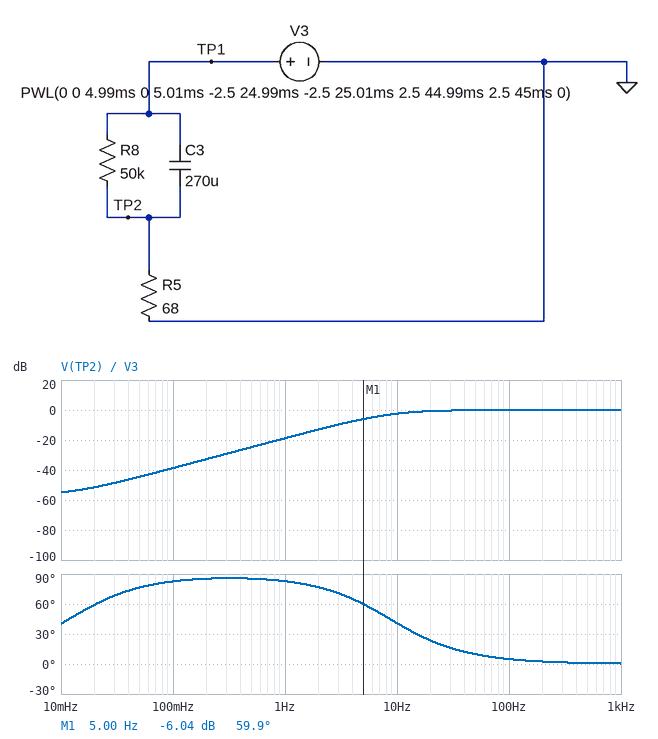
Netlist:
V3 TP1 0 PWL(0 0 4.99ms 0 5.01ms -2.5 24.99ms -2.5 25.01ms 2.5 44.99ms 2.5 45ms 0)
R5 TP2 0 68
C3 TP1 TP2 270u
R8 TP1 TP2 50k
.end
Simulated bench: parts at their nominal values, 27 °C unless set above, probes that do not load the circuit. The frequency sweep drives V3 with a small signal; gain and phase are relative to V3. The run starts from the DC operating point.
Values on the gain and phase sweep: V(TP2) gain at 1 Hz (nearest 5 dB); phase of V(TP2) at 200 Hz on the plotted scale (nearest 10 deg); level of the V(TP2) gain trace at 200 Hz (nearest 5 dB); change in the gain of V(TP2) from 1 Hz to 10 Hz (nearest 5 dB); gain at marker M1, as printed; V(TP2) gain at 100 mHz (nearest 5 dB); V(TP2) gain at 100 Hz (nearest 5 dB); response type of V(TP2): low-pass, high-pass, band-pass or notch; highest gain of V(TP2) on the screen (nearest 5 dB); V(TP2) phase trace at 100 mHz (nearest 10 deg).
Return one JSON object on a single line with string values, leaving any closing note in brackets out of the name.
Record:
{"V(TP2) gain at 1 Hz": "-20 dB", "phase of V(TP2) at 200 Hz on the plotted scale": "0 deg", "level of the V(TP2) gain trace at 200 Hz": "0 dB", "change in the gain of V(TP2) from 1 Hz to 10 Hz": "15 dB", "gain at marker M1, as printed": "-6.04 dB", "V(TP2) gain at 100 mHz": "-40 dB", "V(TP2) gain at 100 Hz": "0 dB", "response type of V(TP2): low-pass, high-pass, band-pass or notch": "high-pass", "highest gain of V(TP2) on the screen": "0 dB", "V(TP2) phase trace at 100 mHz": "80 deg"}
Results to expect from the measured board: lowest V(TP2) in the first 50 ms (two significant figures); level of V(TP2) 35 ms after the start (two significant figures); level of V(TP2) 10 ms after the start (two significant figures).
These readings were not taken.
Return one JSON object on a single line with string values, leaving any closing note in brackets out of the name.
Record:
{"lowest V(TP2) in the first 50 ms": "-2.5 V", "level of V(TP2) 35 ms after the start": "2.4 V", "level of V(TP2) 10 ms after the start": "-1.9 V"}
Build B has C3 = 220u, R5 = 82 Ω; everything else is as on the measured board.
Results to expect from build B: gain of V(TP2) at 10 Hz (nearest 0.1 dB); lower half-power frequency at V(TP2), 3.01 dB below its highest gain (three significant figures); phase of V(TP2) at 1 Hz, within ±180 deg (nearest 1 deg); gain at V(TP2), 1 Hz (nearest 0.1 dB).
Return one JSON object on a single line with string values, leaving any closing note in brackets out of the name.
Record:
{"gain of V(TP2) at 10 Hz": "-2.5 dB", "lower half-power frequency at V(TP2), 3.01 dB below its highest gain": "8.84 Hz", "phase of V(TP2) at 1 Hz, within ±180 deg": "83 deg", "gain at V(TP2), 1 Hz": "-19.0 dB"}
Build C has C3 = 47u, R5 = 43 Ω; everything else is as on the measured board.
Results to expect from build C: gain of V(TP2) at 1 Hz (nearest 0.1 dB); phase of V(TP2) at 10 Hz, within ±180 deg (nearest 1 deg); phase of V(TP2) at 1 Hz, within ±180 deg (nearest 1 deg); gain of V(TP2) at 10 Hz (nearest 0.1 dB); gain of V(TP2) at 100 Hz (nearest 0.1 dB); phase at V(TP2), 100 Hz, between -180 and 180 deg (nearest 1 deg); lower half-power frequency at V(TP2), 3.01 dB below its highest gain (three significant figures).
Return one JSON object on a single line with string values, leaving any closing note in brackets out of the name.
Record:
{"gain of V(TP2) at 1 Hz": "-37.9 dB", "phase of V(TP2) at 10 Hz, within ±180 deg": "82 deg", "phase of V(TP2) at 1 Hz, within ±180 deg": "85 deg", "gain of V(TP2) at 10 Hz": "-18.0 dB", "gain of V(TP2) at 100 Hz": "-2.1 dB", "phase at V(TP2), 100 Hz, between -180 and 180 deg": "38 deg", "lower half-power frequency at V(TP2), 3.01 dB below its highest gain": "78.8 Hz"}
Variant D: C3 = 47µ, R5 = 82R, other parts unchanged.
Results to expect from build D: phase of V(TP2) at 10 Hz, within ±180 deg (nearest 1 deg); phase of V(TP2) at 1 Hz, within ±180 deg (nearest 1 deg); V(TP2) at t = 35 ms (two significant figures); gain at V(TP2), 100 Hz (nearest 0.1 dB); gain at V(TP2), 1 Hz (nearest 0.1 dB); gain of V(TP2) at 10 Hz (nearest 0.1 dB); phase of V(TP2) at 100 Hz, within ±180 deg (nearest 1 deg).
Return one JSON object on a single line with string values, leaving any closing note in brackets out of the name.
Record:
{"phase of V(TP2) at 10 Hz, within ±180 deg": "76 deg", "phase of V(TP2) at 1 Hz, within ±180 deg": "85 deg", "V(TP2) at t = 35 ms": "370 mV", "gain at V(TP2), 100 Hz": "-0.7 dB", "gain at V(TP2), 1 Hz": "-32.3 dB", "gain of V(TP2) at 10 Hz": "-12.6 dB", "phase of V(TP2) at 100 Hz, within ±180 deg": "22 deg"}
